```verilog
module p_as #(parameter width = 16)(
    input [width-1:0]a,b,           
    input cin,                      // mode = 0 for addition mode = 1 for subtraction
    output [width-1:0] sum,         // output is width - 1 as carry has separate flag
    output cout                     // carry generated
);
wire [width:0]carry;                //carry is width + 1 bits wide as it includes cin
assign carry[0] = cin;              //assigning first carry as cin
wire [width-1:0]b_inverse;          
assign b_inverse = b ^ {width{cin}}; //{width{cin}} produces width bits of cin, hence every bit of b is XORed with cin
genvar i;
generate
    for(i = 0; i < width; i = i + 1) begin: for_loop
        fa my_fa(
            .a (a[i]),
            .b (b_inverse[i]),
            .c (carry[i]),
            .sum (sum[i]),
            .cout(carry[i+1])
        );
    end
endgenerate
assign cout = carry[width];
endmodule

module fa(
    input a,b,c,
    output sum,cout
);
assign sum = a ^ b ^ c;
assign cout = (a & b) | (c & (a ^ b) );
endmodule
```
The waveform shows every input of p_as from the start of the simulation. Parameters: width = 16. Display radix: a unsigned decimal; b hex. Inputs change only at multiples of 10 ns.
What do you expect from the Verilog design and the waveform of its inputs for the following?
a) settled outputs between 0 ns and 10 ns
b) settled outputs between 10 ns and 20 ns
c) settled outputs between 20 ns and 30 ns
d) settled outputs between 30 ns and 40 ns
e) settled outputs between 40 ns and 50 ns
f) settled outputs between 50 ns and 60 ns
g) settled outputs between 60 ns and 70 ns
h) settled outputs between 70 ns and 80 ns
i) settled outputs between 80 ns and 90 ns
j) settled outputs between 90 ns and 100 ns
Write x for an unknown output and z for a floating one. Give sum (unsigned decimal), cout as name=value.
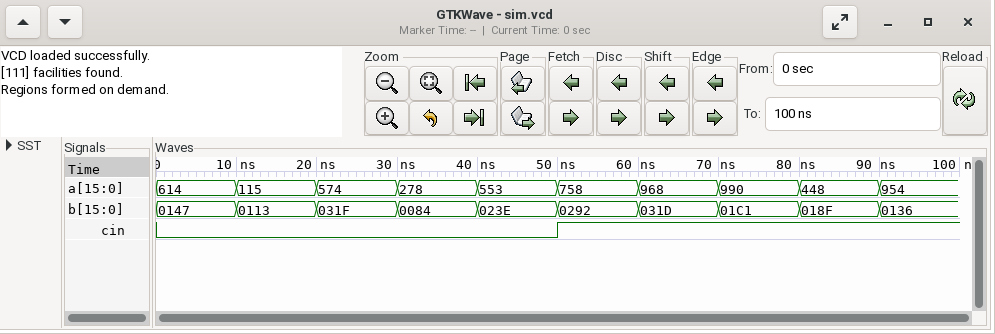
sum=941, cout=0
sum=390, cout=0
sum=1373, cout=0
sum=410, cout=0
sum=1127, cout=0
sum=100, cout=1
sum=171, cout=1
sum=541, cout=1
sum=49, cout=1
sum=644, cout=1
